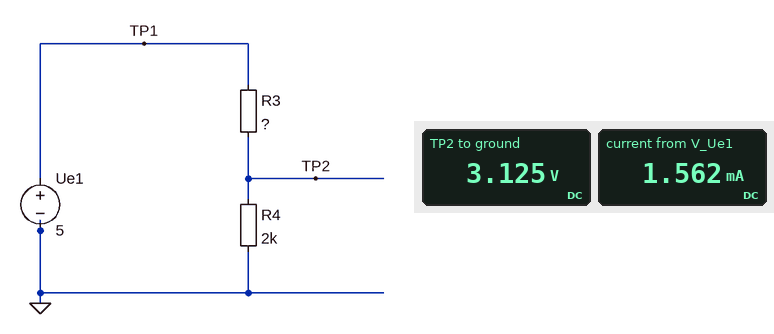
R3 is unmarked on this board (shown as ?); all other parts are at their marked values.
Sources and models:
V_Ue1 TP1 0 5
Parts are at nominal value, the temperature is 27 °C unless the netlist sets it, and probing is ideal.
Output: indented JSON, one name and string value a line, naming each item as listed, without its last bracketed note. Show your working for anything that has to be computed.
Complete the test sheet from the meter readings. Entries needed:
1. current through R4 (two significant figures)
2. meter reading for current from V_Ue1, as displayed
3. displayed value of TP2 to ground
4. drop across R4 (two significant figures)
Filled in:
{
  "current through R4": "(3.125 V) / 2 kΩ = 1.6 mA",
  "meter reading for current from V_Ue1, as displayed": "1.562 mA",
  "displayed value of TP2 to ground": "3.125 V",
  "drop across R4": "3.125 V = 3.1 V"
}
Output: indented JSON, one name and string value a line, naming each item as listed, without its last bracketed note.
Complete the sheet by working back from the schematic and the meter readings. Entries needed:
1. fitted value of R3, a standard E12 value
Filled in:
{
  "fitted value of R3, a standard E12 value": "1.2 kΩ"
}
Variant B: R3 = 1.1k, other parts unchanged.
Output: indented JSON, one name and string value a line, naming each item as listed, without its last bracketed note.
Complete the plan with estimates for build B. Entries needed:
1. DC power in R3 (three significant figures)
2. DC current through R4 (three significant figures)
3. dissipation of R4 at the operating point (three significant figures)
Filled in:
{
  "DC power in R3": "2.86 mW",
  "DC current through R4": "1.61 mA",
  "dissipation of R4 at the operating point": "5.20 mW"
}
